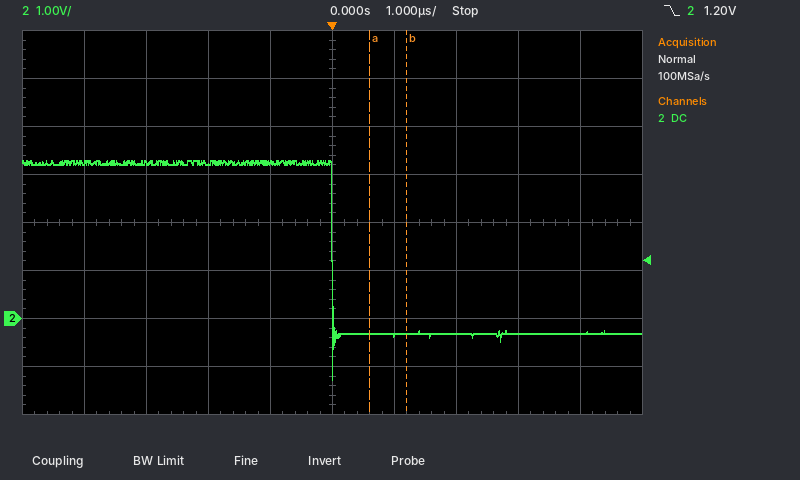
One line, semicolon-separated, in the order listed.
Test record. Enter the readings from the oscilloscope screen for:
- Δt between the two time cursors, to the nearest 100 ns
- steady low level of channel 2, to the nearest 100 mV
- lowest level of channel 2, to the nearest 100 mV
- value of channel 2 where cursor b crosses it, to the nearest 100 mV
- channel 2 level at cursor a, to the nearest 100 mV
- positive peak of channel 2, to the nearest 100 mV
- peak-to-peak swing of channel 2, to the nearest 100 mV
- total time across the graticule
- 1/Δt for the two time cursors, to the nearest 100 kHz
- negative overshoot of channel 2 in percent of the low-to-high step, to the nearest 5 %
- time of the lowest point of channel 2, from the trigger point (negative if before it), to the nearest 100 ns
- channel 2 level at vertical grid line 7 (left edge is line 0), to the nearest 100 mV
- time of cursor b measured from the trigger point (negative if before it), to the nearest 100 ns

600 ns; -300 mV; -1.3 V; -300 mV; -300 mV; 3.3 V; 4.6 V; 10 µs; 1.7 MHz; 25 %; 0.0 µs; -300 mV; +1.2 µs
